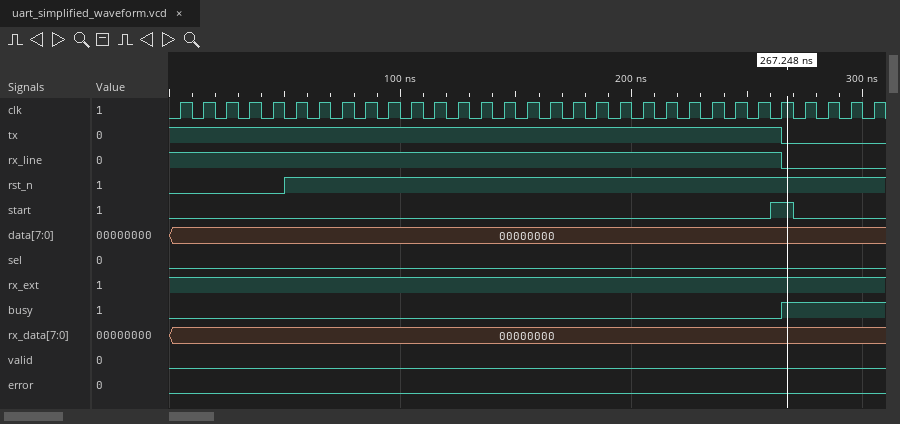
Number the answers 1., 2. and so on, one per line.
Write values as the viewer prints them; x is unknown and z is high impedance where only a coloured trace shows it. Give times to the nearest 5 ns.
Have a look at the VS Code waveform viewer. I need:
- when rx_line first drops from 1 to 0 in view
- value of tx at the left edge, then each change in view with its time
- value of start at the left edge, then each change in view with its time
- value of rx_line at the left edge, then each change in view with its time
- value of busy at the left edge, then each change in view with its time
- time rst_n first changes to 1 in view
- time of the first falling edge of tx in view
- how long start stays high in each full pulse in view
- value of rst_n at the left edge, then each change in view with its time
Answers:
1. 265 ns
2. 1, 0 at 265 ns
3. 0, 1 at 260 ns, 0 at 270 ns
4. 1, 0 at 265 ns
5. 0, 1 at 265 ns
6. 50 ns
7. 265 ns
8. 10 ns
9. 0, 1 at 50 ns
